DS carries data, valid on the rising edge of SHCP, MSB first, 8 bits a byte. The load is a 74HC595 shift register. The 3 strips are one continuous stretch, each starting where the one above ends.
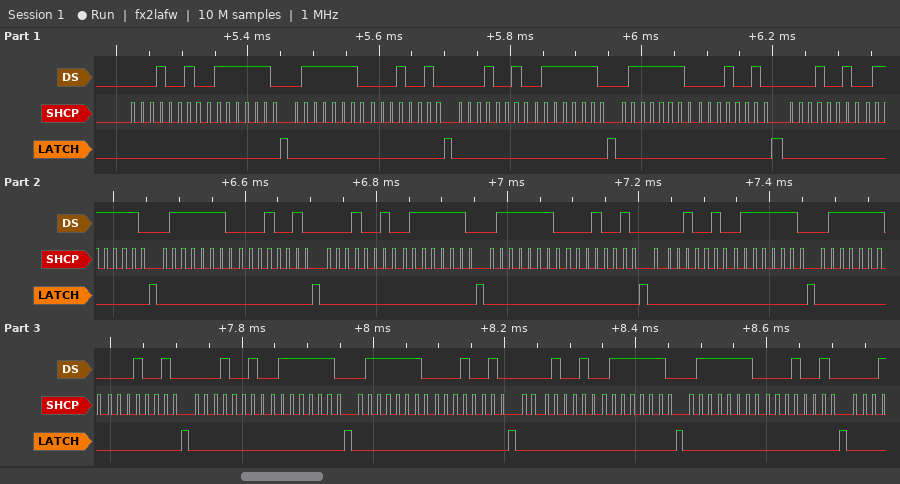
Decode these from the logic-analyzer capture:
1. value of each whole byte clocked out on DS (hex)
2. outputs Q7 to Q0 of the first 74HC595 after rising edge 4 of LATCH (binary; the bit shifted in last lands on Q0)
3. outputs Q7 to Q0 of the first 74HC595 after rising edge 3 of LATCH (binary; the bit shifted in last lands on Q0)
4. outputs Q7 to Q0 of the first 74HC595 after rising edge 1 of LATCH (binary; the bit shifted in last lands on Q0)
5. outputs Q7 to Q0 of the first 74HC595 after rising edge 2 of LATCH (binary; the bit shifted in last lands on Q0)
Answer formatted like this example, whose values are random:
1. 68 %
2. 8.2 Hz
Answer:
1. 12 7E 7E 12 12 7E 7E 12 12 7E 7E 12 12 7E 7E 12 12 7E 7E 12 12 7E 7E 12 12 7E 7E 12
2. 00010010
3. 01111110
4. 01111110
5. 00010010
